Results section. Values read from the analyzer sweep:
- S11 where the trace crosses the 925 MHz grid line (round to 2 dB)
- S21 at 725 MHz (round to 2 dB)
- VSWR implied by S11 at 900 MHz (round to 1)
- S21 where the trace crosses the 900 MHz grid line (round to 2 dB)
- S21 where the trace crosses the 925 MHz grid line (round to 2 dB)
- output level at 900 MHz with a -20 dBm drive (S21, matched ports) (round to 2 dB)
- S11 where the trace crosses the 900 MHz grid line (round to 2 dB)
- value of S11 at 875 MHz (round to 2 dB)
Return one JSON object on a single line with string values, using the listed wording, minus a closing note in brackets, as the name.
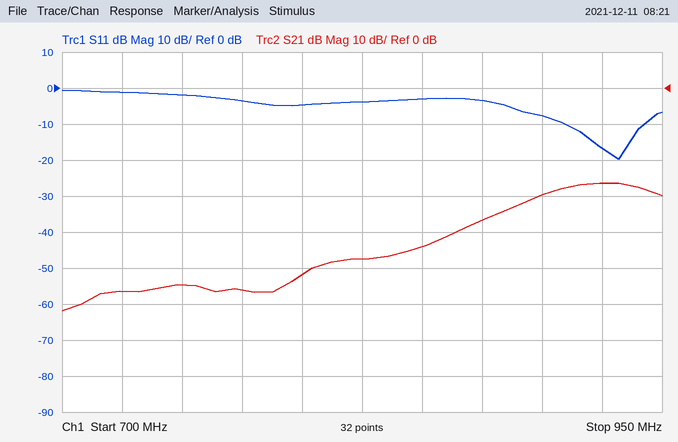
{"S11 where the trace crosses the 925 MHz grid line": "-16 dB", "S21 at 725 MHz": "-56 dB", "VSWR implied by S11 at 900 MHz": "2", "S21 where the trace crosses the 900 MHz grid line": "-30 dB", "S21 where the trace crosses the 925 MHz grid line": "-26 dB", "output level at 900 MHz with a -20 dBm drive (S21, matched ports)": "-50 dBm", "S11 where the trace crosses the 900 MHz grid line": "-8 dB", "value of S11 at 875 MHz": "-4 dB"}
